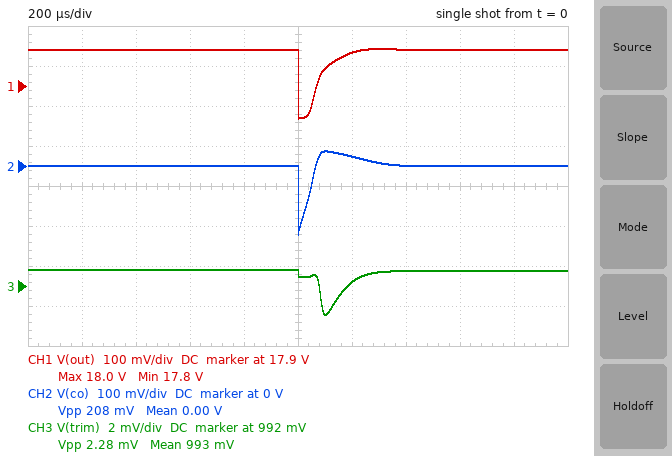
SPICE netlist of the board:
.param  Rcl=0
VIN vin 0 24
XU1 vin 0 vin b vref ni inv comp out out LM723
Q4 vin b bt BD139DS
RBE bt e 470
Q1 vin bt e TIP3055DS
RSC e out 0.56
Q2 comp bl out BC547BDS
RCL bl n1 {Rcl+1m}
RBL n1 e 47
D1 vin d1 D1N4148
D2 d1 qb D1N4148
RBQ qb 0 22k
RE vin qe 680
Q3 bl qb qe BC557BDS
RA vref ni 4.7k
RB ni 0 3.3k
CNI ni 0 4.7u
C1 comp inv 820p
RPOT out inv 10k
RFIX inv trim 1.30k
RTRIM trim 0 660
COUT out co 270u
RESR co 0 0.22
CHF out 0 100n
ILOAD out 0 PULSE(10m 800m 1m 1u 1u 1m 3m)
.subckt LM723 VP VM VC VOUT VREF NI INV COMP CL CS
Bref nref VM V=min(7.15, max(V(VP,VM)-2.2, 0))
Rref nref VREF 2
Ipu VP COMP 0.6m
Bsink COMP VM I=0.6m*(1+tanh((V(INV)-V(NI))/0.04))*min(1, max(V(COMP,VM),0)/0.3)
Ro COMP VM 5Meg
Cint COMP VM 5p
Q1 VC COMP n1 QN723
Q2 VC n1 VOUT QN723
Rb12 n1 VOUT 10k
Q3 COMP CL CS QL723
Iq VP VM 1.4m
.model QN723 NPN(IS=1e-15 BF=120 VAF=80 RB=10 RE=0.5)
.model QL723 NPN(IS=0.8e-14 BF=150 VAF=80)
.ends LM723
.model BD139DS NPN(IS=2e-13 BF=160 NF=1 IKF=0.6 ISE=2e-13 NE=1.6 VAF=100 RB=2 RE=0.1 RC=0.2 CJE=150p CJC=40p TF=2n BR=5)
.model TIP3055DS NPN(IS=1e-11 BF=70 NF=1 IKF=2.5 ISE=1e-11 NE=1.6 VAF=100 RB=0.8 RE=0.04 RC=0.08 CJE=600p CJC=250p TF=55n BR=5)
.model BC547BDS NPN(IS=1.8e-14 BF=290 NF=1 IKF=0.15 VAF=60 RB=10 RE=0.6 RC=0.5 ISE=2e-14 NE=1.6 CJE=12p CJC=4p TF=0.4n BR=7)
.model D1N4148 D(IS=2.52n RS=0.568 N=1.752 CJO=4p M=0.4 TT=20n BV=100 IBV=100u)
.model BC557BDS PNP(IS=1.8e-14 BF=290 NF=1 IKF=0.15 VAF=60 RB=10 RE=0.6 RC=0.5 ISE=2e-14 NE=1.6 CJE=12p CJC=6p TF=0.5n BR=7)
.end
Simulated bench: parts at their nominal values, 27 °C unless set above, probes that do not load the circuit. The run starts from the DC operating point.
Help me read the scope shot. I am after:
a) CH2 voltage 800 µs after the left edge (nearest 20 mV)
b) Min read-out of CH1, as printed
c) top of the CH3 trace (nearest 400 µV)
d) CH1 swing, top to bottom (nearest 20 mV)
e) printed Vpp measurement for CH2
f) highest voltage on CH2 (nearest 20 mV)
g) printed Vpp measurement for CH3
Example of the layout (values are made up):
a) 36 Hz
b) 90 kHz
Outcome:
a) 0 V
b) 17.8 V
c) 992.8 mV
d) 180 mV
e) 208 mV
f) 40 mV
g) 2.28 mV
